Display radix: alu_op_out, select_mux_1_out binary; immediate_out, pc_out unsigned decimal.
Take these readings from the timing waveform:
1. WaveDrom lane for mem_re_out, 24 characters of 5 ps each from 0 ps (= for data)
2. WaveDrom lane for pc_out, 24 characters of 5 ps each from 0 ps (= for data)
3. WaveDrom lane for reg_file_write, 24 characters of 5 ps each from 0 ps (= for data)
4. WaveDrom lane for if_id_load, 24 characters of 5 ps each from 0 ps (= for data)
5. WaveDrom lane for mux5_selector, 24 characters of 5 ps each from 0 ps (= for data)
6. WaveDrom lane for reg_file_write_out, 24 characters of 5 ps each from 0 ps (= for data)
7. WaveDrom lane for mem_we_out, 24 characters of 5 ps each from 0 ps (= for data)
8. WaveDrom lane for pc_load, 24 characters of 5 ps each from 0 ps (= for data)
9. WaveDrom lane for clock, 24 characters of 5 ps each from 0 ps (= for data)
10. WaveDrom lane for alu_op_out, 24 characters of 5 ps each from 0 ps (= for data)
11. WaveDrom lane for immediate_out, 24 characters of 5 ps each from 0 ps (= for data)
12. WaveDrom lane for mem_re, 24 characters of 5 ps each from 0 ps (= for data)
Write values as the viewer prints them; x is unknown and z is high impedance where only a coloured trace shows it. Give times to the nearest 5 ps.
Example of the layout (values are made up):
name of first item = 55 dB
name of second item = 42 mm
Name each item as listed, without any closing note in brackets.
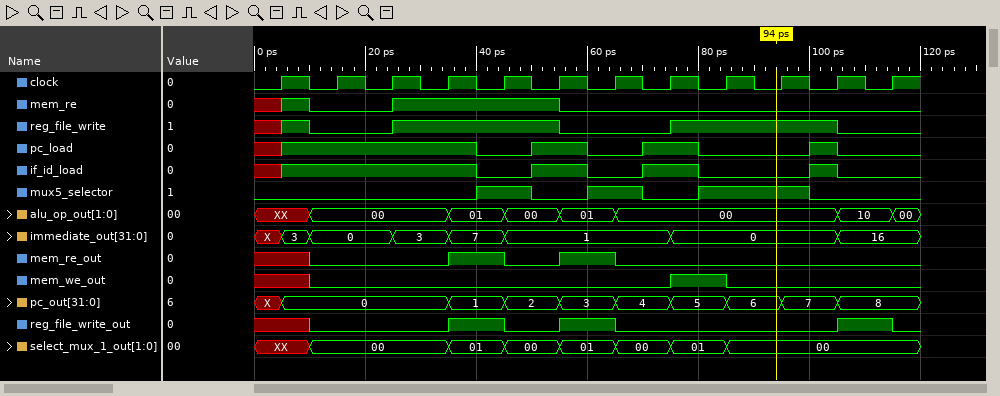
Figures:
WaveDrom lane for mem_re_out, 24 characters of 5 ps each from 0 ps = {name: 'mem_re_out', wave: 'x.0....1.0.1.0..........'}
WaveDrom lane for pc_out, 24 characters of 5 ps each from 0 ps = {name: 'pc_out', wave: 'x=.....=.=.=.=.=.=.=.=..', data: '0 1 2 3 4 5 6 7 8'}
WaveDrom lane for reg_file_write, 24 characters of 5 ps each from 0 ps = {name: 'reg_file_write', wave: 'x10..1.....0...1.....0..'}
WaveDrom lane for if_id_load, 24 characters of 5 ps each from 0 ps = {name: 'if_id_load', wave: 'x1......0.1.0.1.0...10..'}
WaveDrom lane for mux5_selector, 24 characters of 5 ps each from 0 ps = {name: 'mux5_selector', wave: '0.......1.0.1.0.1...0...'}
WaveDrom lane for reg_file_write_out, 24 characters of 5 ps each from 0 ps = {name: 'reg_file_write_out', wave: 'x.0....1.0.1.0.......1.0'}
WaveDrom lane for mem_we_out, 24 characters of 5 ps each from 0 ps = {name: 'mem_we_out', wave: 'x.0............1.0......'}
WaveDrom lane for pc_load, 24 characters of 5 ps each from 0 ps = {name: 'pc_load', wave: 'x1......0.1.0.1.0...10..'}
WaveDrom lane for clock, 24 characters of 5 ps each from 0 ps = {name: 'clock', wave: '010101010101010101010101'}
WaveDrom lane for alu_op_out, 24 characters of 5 ps each from 0 ps = {name: 'alu_op_out', wave: 'x.=....=.=.=.=.......=.=', data: '00 01 00 01 00 10 00'}
WaveDrom lane for immediate_out, 24 characters of 5 ps each from 0 ps = {name: 'immediate_out', wave: 'x==..=.=.=.....=.....=..', data: '3 0 3 7 1 0 16'}
WaveDrom lane for mem_re, 24 characters of 5 ps each from 0 ps = {name: 'mem_re', wave: 'x10..1.....0............'}
